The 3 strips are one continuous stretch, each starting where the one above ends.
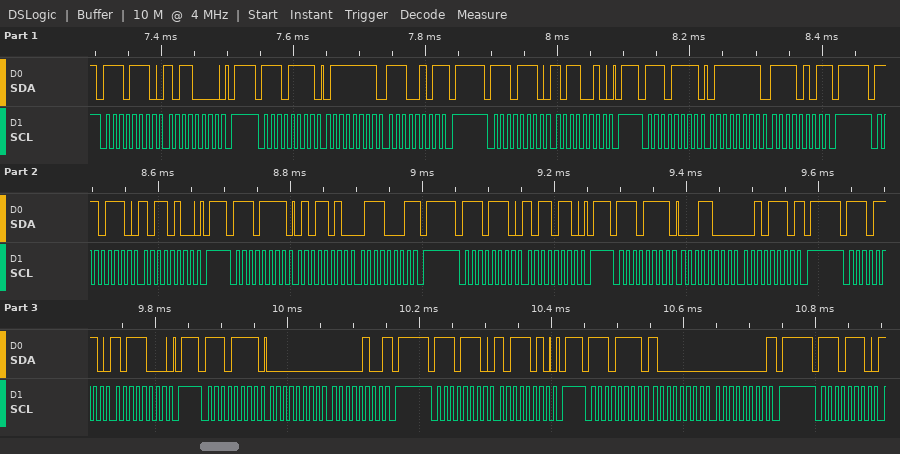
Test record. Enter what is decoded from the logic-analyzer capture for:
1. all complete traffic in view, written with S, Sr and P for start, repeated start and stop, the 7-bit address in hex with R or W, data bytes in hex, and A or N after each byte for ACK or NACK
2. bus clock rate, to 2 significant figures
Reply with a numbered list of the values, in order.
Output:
1. S 77W A B0 A P S 77R A 7F A E5 N P S 77W A B2 A P S 77R A 7F A F5 N P S 77W A B4 A P S 77R A 5A A 71 N P S 77W A B6 A P S 77R A 18 A 2E N P S 77W A B8 A P S 77R A 00 A 04 N P S 77W A BA A P S 77R A 80 A 00 N P S 77W A
2. 100 kHz
